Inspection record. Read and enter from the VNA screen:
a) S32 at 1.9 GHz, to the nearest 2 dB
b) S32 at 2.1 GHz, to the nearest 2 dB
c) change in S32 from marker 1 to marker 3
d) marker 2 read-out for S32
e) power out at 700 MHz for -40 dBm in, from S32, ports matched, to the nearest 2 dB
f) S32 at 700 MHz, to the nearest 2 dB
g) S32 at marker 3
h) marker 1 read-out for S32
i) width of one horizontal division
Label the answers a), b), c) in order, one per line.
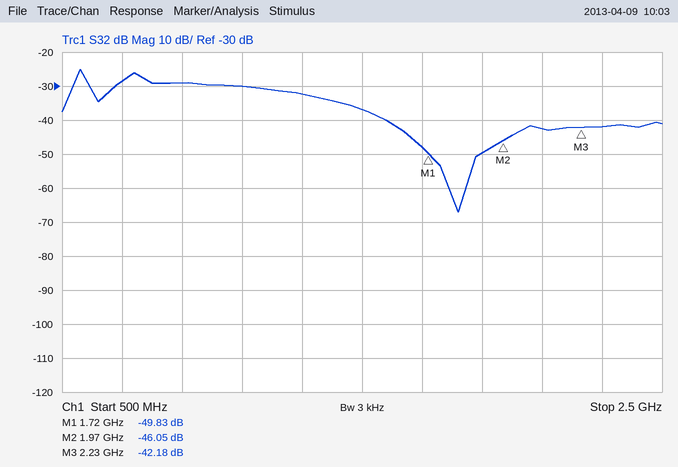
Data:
a) -50 dB
b) -42 dB
c) 7.65 dB
d) -46.05 dB
e) -68 dBm
f) -28 dB
g) -42.18 dB
h) -49.83 dB
i) 200 MHz
